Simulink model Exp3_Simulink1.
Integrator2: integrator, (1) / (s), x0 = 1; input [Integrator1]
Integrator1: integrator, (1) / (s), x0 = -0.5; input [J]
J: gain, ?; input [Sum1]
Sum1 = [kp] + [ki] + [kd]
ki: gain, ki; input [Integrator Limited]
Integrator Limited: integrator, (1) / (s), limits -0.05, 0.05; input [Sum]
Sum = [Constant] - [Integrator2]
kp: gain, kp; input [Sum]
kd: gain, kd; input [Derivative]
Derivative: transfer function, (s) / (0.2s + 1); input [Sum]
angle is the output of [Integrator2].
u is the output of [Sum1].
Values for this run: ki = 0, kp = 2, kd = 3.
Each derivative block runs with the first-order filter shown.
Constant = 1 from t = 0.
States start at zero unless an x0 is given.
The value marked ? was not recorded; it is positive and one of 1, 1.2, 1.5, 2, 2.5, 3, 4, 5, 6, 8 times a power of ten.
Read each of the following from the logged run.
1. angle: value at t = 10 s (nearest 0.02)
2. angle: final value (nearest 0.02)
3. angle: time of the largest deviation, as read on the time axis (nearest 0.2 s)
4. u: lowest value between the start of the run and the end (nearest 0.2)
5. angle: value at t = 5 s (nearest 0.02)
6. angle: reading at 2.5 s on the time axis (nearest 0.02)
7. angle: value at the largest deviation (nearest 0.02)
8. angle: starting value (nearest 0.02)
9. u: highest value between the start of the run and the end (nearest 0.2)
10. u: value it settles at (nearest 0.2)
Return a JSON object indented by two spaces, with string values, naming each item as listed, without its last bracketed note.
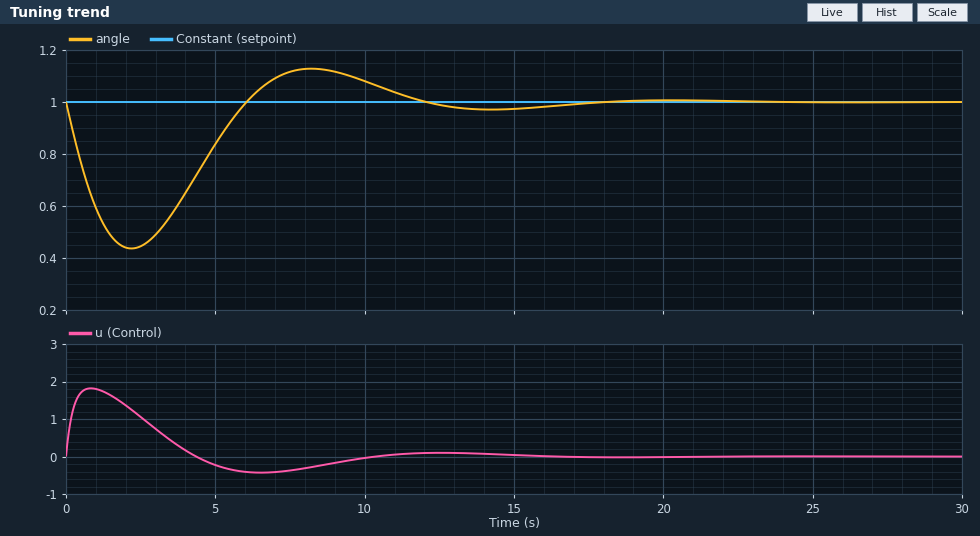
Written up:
{
  "angle: value at t = 10 s": "1.08",
  "angle: final value": "1.00",
  "angle: time of the largest deviation, as read on the time axis": "2.2 s",
  "u: lowest value between the start of the run and the end": "-0.4",
  "angle: value at t = 5 s": "0.84",
  "angle: reading at 2.5 s on the time axis": "0.44",
  "angle: value at the largest deviation": "0.44",
  "angle: starting value": "1.00",
  "u: highest value between the start of the run and the end": "1.8",
  "u: value it settles at": "0.0"
}
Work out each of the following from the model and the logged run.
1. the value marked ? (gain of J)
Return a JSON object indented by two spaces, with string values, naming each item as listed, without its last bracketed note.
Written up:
{
  "the value marked ?": "0.15"
}
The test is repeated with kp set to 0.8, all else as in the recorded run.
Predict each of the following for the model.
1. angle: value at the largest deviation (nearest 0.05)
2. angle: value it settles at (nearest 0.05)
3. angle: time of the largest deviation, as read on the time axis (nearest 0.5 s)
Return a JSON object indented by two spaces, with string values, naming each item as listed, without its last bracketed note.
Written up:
{
  "angle: value at the largest deviation": "0.30",
  "angle: value it settles at": "1.00",
  "angle: time of the largest deviation, as read on the time axis": "3.0 s"
}
